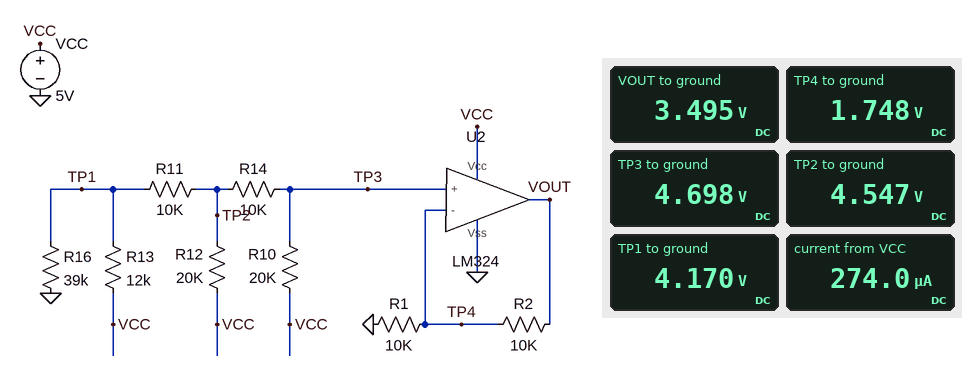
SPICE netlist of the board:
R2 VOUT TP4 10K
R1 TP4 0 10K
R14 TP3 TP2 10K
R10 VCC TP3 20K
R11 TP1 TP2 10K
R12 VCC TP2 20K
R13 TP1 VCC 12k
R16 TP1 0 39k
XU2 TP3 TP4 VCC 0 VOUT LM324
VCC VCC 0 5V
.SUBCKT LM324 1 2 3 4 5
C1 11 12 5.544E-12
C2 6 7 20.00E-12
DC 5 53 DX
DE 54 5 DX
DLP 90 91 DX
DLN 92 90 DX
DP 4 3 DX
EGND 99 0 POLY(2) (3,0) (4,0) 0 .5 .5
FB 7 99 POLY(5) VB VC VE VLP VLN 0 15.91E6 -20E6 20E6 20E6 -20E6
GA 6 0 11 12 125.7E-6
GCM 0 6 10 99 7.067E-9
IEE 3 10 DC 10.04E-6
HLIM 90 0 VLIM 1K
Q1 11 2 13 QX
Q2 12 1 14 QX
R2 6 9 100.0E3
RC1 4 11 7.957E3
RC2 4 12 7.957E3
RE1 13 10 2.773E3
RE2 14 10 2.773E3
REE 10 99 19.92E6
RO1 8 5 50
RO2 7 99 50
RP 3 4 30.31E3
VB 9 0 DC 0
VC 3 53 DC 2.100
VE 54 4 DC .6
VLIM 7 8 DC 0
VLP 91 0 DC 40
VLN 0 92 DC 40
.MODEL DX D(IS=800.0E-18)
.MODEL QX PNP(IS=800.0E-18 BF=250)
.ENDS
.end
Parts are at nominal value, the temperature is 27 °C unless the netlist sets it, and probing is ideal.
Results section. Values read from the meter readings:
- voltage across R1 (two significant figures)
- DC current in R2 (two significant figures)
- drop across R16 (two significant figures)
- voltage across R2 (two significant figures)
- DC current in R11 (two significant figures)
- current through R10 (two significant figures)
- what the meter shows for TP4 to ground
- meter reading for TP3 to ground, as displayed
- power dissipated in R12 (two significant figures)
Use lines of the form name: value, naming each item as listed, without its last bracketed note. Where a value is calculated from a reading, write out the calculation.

voltage across R1: 1.748 V = 1.7 V
DC current in R2: (3.495 V - 1.748 V) / 10 kΩ = 170 µA
drop across R16: 4.17 V = 4.2 V
voltage across R2: 3.495 V - 1.748 V = 1.7 V
DC current in R11: (4.547 V - 4.17 V) / 10 kΩ = 38 µA
current through R10: (5 V - 4.698 V) / 20 kΩ = 15 µA
what the meter shows for TP4 to ground: 1.748 V
meter reading for TP3 to ground, as displayed: 4.698 V
power dissipated in R12: (5 V - 4.547 V)^2 / 20 kΩ = 10 µW
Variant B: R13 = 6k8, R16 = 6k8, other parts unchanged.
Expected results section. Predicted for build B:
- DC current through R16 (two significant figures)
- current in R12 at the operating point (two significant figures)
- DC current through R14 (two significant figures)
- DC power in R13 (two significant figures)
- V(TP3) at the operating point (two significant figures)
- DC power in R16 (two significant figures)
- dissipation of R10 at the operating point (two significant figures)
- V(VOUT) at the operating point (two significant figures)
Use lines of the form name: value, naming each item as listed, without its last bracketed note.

DC current through R16: 420 µA
current in R12 at the operating point: 59 µA
DC current through R14: 39 µA
DC power in R13: 690 µW
V(TP3) at the operating point: 4.2 V
DC power in R16: 1.2 mW
dissipation of R10 at the operating point: 31 µW
V(VOUT) at the operating point: 3.5 V
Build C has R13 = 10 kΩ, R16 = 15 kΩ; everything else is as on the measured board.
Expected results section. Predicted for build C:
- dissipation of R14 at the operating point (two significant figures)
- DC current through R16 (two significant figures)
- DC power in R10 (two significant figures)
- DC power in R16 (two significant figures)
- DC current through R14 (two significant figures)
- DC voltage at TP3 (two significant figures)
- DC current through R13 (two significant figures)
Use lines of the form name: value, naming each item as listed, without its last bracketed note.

dissipation of R14 at the operating point: 8.2 µW
DC current through R16: 230 µA
DC power in R10: 16 µW
DC power in R16: 780 µW
DC current through R14: 29 µA
DC voltage at TP3: 4.4 V
DC current through R13: 160 µA
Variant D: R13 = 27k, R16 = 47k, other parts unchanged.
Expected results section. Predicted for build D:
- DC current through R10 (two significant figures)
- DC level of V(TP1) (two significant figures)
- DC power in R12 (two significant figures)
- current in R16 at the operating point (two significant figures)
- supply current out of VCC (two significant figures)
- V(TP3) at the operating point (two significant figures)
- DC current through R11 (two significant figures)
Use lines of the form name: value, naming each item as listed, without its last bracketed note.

DC current through R10: 19 µA
DC level of V(TP1): 4.0 V
DC power in R12: 16 µW
current in R16 at the operating point: 85 µA
supply current out of VCC: 250 µA
V(TP3) at the operating point: 4.6 V
DC current through R11: 47 µA
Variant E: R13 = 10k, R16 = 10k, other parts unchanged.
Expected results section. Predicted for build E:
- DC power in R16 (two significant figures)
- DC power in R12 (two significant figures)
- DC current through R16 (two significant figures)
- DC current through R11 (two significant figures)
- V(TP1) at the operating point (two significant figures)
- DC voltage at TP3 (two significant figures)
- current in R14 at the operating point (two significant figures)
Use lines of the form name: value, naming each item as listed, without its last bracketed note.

DC power in R16: 880 µW
DC power in R12: 62 µW
DC current through R16: 300 µA
DC current through R11: 93 µA
V(TP1) at the operating point: 3.0 V
DC voltage at TP3: 4.3 V
current in R14 at the operating point: 37 µA
